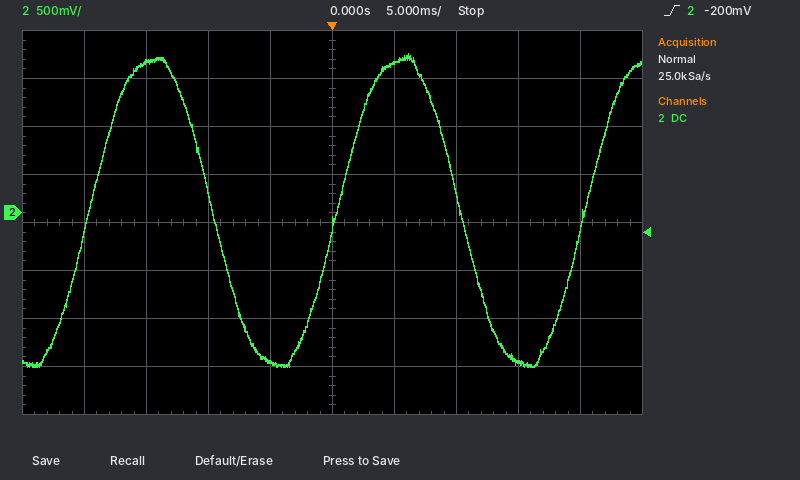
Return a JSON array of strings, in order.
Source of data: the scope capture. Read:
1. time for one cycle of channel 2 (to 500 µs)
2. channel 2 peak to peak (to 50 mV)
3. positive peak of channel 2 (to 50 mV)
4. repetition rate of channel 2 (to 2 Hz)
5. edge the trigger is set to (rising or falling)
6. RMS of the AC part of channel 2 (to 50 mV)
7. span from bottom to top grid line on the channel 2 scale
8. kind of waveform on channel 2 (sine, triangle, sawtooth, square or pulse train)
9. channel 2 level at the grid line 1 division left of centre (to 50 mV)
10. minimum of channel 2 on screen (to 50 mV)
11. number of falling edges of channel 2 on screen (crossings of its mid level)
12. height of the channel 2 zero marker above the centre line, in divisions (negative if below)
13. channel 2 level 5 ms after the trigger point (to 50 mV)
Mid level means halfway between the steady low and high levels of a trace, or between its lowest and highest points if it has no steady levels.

["20.0 ms", "3.25 V", "1.65 V", "50 Hz", "rising", "1.15 V", "4 V", "sine", "-1.55 V", "-1.60 V", "2", "+0.2 div", "1.55 V"]
